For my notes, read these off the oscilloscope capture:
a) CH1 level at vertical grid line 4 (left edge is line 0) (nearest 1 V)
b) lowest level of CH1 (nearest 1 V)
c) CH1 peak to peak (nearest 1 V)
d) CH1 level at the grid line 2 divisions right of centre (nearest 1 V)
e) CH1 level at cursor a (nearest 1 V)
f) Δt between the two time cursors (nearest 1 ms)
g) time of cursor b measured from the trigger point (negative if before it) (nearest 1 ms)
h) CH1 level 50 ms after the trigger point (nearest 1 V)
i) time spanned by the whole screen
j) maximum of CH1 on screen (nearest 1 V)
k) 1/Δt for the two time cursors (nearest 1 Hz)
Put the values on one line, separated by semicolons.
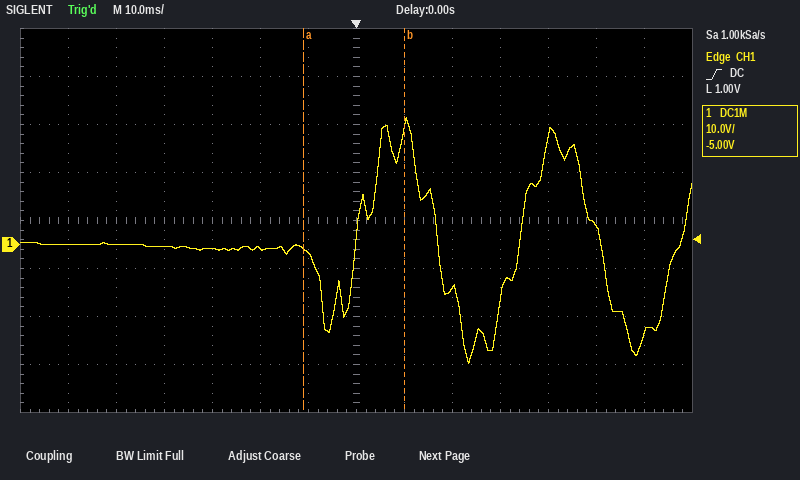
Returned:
-1 V; -25 V; 51 V; -9 V; -1 V; 21 ms; +10 ms; 4 V; 140 ms; 26 V; 48 Hz
